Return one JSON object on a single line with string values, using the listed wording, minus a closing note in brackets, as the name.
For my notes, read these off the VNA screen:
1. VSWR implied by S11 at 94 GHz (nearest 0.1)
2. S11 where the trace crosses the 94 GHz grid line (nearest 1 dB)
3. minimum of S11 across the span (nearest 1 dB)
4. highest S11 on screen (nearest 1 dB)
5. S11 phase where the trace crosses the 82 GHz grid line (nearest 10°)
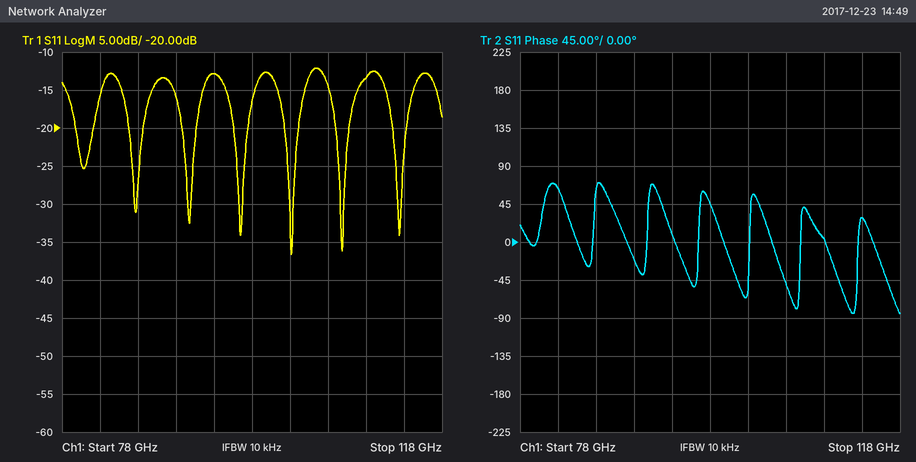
{"VSWR implied by S11 at 94 GHz": "1.6", "S11 where the trace crosses the 94 GHz grid line": "-13 dB", "minimum of S11 across the span": "-37 dB", "highest S11 on screen": "-12 dB", "S11 phase where the trace crosses the 82 GHz grid line": "60°"}
